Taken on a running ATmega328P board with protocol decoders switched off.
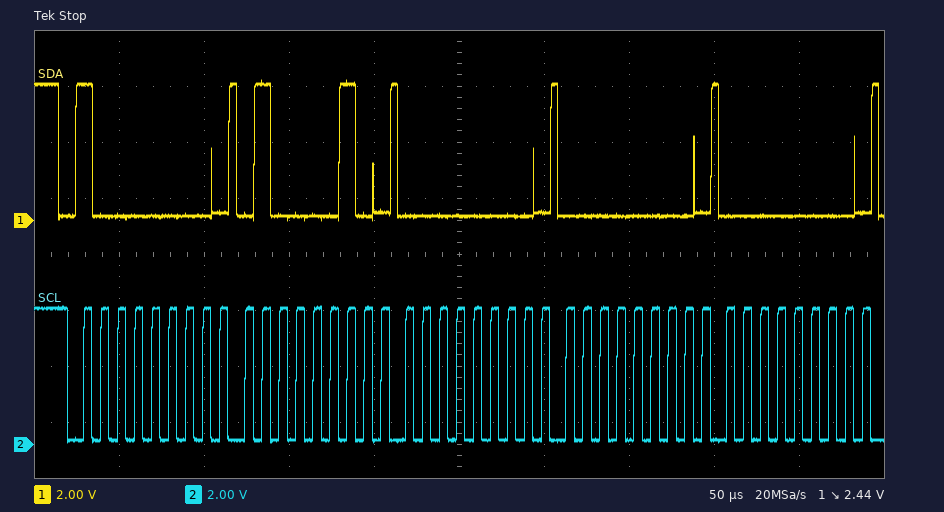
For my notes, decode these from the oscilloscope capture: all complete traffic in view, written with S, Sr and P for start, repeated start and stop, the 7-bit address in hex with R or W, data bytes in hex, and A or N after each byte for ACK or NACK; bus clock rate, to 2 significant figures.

S 40W A 42 A 00 A 00 A 00 A
100 kHz
